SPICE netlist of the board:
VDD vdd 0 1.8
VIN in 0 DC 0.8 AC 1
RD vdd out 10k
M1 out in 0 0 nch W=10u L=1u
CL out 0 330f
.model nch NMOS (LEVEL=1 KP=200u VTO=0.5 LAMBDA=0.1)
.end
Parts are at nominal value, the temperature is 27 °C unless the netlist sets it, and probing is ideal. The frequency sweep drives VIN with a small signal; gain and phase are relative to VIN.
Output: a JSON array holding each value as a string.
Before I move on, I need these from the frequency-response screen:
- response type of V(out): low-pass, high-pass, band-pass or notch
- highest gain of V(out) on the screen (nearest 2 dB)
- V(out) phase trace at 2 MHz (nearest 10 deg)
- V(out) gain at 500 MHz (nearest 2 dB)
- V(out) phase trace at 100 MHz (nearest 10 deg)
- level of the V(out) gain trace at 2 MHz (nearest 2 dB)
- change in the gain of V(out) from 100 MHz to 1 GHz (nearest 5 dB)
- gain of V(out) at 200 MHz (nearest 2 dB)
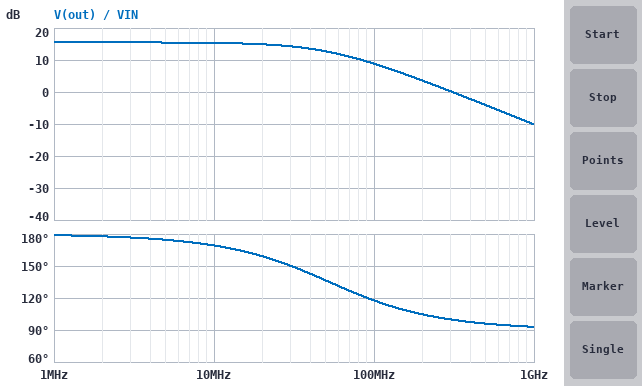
["low-pass", "16 dB", "180 deg", "-4 dB", "120 deg", "16 dB", "-20 dB", "4 dB"]
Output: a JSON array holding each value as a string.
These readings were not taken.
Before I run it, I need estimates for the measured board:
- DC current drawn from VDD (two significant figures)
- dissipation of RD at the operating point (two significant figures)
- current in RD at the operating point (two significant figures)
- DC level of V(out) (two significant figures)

["97 µA", "95 µW", "97 µA", "830 mV"]
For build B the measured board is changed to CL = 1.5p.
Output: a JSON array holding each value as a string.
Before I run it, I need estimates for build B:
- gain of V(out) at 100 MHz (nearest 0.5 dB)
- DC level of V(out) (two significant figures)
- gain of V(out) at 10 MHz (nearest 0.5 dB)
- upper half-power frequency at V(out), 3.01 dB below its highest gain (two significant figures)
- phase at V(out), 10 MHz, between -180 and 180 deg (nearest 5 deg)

["-3.5 dB", "830 mV", "13.0 dB", "12 MHz", "140 deg"]
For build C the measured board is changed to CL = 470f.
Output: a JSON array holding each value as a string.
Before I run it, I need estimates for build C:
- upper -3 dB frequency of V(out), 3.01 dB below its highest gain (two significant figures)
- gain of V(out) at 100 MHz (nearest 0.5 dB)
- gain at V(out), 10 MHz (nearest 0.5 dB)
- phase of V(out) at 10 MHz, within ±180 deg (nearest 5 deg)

["37 MHz", "6.5 dB", "15.0 dB", "165 deg"]
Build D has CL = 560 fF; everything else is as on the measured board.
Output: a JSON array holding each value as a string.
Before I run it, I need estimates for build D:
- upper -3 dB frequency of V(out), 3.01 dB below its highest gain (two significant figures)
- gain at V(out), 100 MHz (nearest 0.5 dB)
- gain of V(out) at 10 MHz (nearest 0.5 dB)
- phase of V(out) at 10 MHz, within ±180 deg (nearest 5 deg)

["31 MHz", "5.0 dB", "15.0 dB", "160 deg"]
